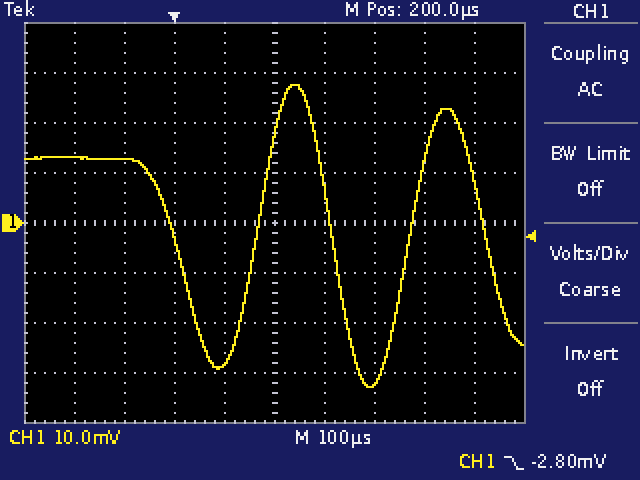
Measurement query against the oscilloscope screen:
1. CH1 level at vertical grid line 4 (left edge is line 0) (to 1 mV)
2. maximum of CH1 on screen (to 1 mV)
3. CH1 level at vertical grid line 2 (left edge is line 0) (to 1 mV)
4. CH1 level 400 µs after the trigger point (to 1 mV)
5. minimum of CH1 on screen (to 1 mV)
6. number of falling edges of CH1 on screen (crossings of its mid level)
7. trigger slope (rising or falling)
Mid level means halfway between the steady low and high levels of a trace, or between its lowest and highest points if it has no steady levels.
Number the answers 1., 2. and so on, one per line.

1. -28 mV
2. 28 mV
3. 13 mV
4. -32 mV
5. -33 mV
6. 3
7. falling
